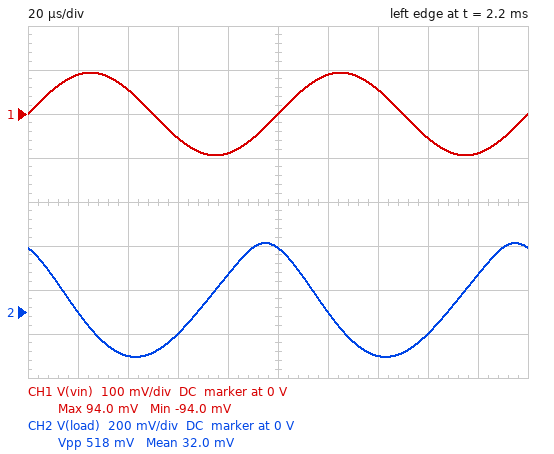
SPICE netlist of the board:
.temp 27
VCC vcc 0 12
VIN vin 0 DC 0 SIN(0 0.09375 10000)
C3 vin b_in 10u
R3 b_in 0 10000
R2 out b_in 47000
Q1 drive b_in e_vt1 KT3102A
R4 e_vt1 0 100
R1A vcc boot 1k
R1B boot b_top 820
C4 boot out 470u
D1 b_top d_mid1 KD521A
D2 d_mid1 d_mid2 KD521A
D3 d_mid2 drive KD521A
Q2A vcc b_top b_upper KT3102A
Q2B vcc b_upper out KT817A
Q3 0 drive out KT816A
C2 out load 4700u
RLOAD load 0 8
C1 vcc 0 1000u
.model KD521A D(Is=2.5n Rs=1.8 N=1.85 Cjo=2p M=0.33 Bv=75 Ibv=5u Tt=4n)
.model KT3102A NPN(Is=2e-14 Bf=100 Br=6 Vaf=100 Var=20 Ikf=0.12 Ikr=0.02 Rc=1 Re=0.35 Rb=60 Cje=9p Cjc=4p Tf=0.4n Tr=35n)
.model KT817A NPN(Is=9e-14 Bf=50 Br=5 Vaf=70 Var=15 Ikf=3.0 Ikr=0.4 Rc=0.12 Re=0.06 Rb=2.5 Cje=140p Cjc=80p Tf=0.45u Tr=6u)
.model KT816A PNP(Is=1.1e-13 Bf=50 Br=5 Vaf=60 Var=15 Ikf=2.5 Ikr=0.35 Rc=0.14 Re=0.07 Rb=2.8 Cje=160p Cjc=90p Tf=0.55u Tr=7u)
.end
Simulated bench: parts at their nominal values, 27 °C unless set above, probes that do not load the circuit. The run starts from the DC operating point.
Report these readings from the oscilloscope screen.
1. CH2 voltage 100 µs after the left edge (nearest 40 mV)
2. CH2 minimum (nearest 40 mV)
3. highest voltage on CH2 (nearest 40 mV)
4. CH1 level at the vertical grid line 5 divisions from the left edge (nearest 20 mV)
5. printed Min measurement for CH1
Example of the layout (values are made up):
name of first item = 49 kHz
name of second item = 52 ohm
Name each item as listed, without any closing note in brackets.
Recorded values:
CH2 voltage 100 µs after the left edge = 280 mV
CH2 minimum = -200 mV
highest voltage on CH2 = 320 mV
CH1 level at the vertical grid line 5 divisions from the left edge = 0 V
printed Min measurement for CH1 = -94.0 mV
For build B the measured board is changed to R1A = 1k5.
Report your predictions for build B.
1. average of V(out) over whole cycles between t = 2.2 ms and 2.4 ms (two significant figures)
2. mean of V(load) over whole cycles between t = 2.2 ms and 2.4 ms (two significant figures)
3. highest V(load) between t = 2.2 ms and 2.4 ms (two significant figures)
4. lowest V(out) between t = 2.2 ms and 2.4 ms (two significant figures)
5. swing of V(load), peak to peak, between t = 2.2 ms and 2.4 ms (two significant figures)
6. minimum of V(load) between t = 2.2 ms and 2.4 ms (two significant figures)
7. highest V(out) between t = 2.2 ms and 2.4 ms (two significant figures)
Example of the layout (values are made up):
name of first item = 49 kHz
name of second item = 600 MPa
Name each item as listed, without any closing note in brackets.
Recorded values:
average of V(out) over whole cycles between t = 2.2 ms and 2.4 ms = 6.3 V
mean of V(load) over whole cycles between t = 2.2 ms and 2.4 ms = 73 mV
highest V(load) between t = 2.2 ms and 2.4 ms = 480 mV
lowest V(out) between t = 2.2 ms and 2.4 ms = 6.0 V
swing of V(load), peak to peak, between t = 2.2 ms and 2.4 ms = 670 mV
minimum of V(load) between t = 2.2 ms and 2.4 ms = -190 mV
highest V(out) between t = 2.2 ms and 2.4 ms = 6.7 V
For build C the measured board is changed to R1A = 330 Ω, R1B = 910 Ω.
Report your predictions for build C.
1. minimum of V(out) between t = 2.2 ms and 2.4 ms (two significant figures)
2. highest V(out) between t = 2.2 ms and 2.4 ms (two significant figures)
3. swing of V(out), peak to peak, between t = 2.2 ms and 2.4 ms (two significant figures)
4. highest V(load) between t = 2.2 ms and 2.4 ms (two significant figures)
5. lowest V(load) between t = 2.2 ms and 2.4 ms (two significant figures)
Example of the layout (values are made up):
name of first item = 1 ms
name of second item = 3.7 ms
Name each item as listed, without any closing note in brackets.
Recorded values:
minimum of V(out) between t = 2.2 ms and 2.4 ms = 7.1 V
highest V(out) between t = 2.2 ms and 2.4 ms = 7.6 V
swing of V(out), peak to peak, between t = 2.2 ms and 2.4 ms = 490 mV
highest V(load) between t = 2.2 ms and 2.4 ms = 270 mV
lowest V(load) between t = 2.2 ms and 2.4 ms = -210 mV
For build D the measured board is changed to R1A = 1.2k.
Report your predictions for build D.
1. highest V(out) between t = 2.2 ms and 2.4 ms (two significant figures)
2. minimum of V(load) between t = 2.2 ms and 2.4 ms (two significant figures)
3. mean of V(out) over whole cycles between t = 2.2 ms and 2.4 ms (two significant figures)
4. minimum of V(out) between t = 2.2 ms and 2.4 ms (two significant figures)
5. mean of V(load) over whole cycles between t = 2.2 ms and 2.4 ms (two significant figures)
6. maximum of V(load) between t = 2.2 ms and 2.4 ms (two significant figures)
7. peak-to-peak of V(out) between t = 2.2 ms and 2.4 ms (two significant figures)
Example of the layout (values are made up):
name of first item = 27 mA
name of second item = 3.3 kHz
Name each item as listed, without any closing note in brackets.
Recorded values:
highest V(out) between t = 2.2 ms and 2.4 ms = 6.8 V
minimum of V(load) between t = 2.2 ms and 2.4 ms = -200 mV
mean of V(out) over whole cycles between t = 2.2 ms and 2.4 ms = 6.5 V
minimum of V(out) between t = 2.2 ms and 2.4 ms = 6.2 V
mean of V(load) over whole cycles between t = 2.2 ms and 2.4 ms = 41 mV
maximum of V(load) between t = 2.2 ms and 2.4 ms = 350 mV
peak-to-peak of V(out) between t = 2.2 ms and 2.4 ms = 550 mV
